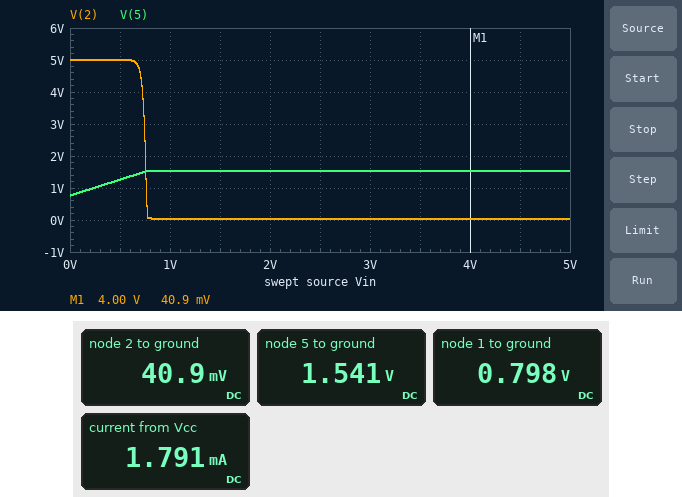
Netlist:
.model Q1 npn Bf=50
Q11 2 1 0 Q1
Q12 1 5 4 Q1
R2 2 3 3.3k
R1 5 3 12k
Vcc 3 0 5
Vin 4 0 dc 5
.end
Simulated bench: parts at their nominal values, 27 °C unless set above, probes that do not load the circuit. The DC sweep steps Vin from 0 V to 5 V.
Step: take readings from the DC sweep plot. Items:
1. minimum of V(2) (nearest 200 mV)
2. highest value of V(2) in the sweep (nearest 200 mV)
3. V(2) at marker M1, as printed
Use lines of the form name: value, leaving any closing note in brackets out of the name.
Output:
minimum of V(2): 0 V
highest value of V(2) in the sweep: 5.0 V
V(2) at marker M1, as printed: 40.9 mV
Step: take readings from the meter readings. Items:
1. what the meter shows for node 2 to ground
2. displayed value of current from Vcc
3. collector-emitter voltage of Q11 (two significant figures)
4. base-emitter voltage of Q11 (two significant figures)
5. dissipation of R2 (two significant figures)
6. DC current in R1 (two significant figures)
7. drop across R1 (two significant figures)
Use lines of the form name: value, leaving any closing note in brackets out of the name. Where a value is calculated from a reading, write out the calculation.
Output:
what the meter shows for node 2 to ground: 40.9 mV
displayed value of current from Vcc: 1.791 mA
collector-emitter voltage of Q11: 40.9 mV = 41 mV
base-emitter voltage of Q11: 798 mV = 800 mV
dissipation of R2: (5 V - 40.9 mV)^2 / 3.3 kΩ = 7.5 mW
DC current in R1: (5 V - 1.541 V) / 12 kΩ = 290 µA
drop across R1: 5 V - 1.541 V = 3.5 V
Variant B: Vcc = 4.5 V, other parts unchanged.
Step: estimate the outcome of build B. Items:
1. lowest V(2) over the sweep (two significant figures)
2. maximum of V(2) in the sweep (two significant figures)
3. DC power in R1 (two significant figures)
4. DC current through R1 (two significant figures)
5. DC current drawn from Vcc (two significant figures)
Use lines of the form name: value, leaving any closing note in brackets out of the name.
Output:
lowest V(2) over the sweep: 42 mV
maximum of V(2) in the sweep: 4.5 V
DC power in R1: 730 µW
DC current through R1: 250 µA
DC current drawn from Vcc: 1.6 mA
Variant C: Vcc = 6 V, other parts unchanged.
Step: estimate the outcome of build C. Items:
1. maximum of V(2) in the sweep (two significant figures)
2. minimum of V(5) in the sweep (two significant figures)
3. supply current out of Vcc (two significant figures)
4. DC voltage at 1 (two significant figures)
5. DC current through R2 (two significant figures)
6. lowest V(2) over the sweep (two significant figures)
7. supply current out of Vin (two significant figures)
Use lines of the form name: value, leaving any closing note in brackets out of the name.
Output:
maximum of V(2) in the sweep: 6.0 V
minimum of V(5) in the sweep: 770 mV
supply current out of Vcc: 2.2 mA
DC voltage at 1: 800 mV
DC current through R2: 1.8 mA
lowest V(2) over the sweep: 40 mV
supply current out of Vin: 370 µA
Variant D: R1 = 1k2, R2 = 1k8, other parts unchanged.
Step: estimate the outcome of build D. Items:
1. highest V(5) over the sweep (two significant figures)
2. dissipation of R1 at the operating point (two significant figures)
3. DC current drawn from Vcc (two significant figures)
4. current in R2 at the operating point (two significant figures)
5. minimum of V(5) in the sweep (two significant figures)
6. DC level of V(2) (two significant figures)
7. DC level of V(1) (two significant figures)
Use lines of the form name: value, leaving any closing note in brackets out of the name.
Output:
highest V(5) over the sweep: 1.6 V
dissipation of R1 at the operating point: 9.4 mW
DC current drawn from Vcc: 5.6 mA
current in R2 at the operating point: 2.8 mA
minimum of V(5) in the sweep: 820 mV
DC level of V(2): 24 mV
DC level of V(1): 840 mV
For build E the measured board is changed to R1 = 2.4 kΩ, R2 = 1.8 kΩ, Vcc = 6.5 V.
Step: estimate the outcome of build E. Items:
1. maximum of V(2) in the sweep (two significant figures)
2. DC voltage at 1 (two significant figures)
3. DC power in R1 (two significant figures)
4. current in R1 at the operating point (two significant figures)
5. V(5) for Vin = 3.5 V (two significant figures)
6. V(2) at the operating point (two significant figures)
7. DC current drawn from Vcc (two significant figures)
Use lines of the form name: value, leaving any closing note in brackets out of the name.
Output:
maximum of V(2) in the sweep: 6.5 V
DC voltage at 1: 840 mV
DC power in R1: 9.9 mW
current in R1 at the operating point: 2.0 mA
V(5) for Vin = 3.5 V: 1.6 V
V(2) at the operating point: 28 mV
DC current drawn from Vcc: 5.6 mA
